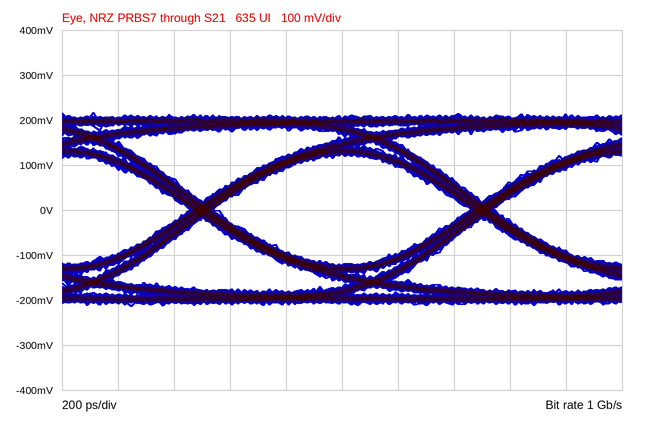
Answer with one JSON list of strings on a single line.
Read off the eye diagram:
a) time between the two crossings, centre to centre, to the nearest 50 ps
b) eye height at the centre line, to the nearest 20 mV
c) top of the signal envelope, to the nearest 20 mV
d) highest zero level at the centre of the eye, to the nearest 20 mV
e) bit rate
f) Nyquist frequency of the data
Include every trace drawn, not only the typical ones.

["1.00 ns", "240 mV", "220 mV", "-120 mV", "1 Gb/s", "500 MHz"]
